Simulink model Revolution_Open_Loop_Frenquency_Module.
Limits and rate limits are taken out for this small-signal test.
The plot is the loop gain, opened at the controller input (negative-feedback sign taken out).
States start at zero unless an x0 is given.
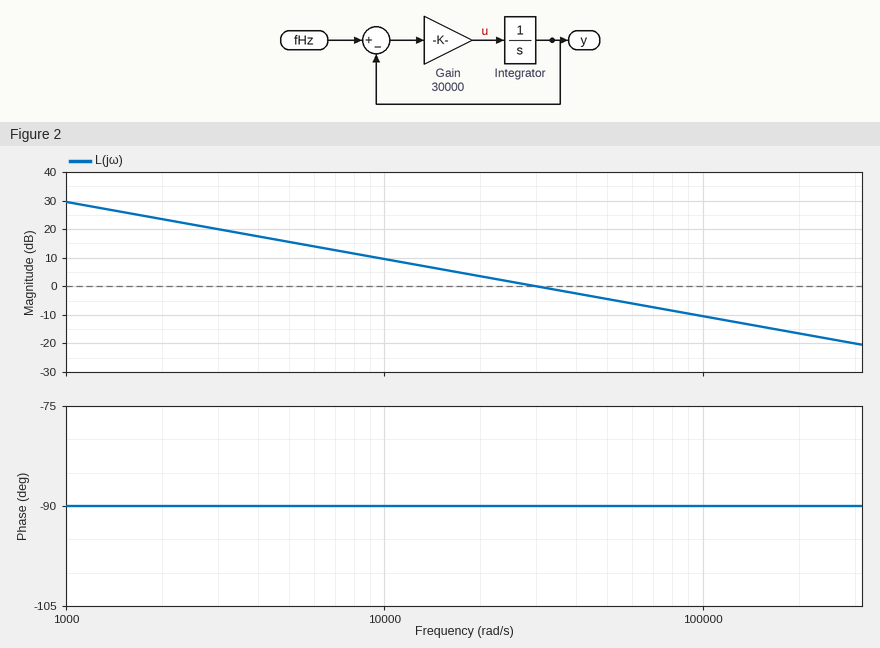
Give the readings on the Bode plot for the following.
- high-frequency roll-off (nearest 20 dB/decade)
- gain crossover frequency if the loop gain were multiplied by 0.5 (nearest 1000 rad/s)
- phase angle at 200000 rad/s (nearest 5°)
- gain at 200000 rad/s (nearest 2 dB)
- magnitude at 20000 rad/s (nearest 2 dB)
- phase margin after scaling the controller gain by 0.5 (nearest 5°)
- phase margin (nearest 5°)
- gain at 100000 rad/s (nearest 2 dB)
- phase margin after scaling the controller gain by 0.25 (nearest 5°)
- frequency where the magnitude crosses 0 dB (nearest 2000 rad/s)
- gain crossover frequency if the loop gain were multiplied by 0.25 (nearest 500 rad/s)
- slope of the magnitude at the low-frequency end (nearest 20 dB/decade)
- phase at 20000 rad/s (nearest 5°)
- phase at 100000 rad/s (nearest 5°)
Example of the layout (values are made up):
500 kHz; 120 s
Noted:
-20 dB/decade; 15000 rad/s; -90°; -16 dB; 4 dB; 90°; 90°; -10 dB; 90°; 30000 rad/s; 7500 rad/s; -20 dB/decade; -90°; -90°
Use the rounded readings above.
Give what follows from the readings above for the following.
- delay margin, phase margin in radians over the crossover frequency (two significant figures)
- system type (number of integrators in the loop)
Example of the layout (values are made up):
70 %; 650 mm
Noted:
0.000052 s; 1
